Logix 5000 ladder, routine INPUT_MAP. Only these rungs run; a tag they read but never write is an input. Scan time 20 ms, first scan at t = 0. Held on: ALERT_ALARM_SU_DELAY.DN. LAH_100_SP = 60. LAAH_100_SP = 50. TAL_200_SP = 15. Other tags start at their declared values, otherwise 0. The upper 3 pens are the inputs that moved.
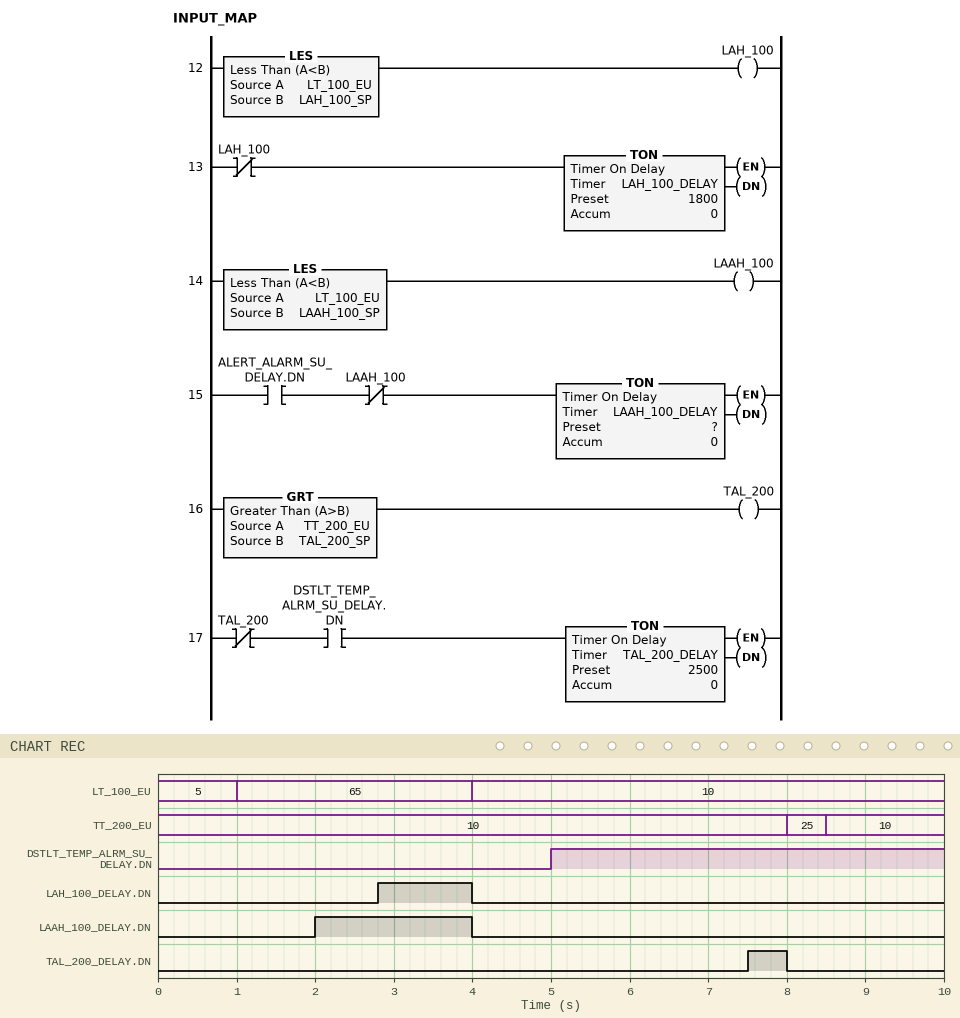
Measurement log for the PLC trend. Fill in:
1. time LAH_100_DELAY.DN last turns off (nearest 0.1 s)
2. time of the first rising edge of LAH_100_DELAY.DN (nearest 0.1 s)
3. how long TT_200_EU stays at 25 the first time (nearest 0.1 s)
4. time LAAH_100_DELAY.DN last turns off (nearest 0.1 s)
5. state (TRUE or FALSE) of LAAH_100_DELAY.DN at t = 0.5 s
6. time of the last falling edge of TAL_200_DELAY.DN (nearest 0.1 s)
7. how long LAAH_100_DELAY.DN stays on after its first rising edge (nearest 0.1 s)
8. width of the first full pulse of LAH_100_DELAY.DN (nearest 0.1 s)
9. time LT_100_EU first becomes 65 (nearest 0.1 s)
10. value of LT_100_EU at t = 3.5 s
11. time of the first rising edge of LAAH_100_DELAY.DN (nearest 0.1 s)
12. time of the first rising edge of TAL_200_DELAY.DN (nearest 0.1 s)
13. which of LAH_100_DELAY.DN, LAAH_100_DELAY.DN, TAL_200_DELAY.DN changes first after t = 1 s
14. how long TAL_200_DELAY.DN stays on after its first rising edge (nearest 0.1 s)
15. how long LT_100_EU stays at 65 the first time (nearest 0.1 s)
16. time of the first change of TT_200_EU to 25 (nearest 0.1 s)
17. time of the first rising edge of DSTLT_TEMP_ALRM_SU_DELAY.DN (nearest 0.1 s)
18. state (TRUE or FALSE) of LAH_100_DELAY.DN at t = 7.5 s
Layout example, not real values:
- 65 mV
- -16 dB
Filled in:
- 4.0 s
- 2.8 s
- 0.5 s
- 4.0 s
- FALSE
- 8.0 s
- 2.0 s
- 1.2 s
- 1.0 s
- 65
- 2.0 s
- 7.5 s
- LAAH_100_DELAY.DN
- 0.5 s
- 3.0 s
- 8.0 s
- 5.0 s
- FALSE
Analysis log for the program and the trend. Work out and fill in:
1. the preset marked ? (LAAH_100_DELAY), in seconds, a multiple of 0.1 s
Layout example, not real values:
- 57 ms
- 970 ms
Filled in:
- 1.0 s
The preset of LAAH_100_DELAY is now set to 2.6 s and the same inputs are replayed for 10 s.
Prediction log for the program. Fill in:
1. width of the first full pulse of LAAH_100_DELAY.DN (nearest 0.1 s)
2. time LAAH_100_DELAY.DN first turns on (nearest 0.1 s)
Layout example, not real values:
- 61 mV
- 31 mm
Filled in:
- 0.4 s
- 3.6 s
